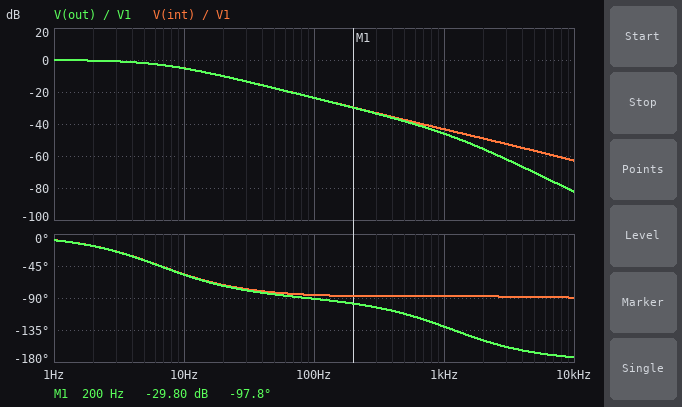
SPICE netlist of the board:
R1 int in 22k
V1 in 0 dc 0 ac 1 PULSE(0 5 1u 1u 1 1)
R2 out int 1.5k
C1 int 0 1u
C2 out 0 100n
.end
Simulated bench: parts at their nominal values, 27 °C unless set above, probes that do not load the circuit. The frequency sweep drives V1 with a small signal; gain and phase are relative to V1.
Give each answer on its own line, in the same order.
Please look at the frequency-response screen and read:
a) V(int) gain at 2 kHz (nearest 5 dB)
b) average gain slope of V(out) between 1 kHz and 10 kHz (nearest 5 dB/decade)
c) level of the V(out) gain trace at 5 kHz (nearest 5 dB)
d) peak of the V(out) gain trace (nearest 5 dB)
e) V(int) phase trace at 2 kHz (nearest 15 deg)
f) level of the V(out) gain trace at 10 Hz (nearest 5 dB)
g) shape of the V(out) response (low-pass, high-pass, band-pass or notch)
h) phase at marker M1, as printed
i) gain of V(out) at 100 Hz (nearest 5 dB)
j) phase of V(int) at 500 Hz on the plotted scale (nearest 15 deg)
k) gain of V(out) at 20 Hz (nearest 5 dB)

-50 dB
-35 dB/decade
-70 dB
0 dB
-90 deg
-5 dB
low-pass
-97.8 deg
-25 dB
-90 deg
-10 dB
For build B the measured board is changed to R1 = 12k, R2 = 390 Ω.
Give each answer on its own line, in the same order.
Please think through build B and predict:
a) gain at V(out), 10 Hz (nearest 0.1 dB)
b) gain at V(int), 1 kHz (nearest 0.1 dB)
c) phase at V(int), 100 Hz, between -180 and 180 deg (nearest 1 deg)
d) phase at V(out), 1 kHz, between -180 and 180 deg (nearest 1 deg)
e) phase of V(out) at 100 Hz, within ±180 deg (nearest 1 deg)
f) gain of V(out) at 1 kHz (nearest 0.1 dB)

-2.3 dB
-38.3 dB
-83 deg
-102 deg
-84 deg
-38.6 dB
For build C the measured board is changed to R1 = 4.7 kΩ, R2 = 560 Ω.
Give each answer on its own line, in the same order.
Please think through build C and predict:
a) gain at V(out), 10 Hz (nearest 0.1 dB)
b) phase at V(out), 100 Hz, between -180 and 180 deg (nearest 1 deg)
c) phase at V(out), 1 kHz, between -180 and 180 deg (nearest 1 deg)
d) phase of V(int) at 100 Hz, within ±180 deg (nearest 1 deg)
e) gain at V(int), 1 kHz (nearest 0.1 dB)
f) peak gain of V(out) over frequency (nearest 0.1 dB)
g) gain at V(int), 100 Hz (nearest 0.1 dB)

-0.4 dB
-75 deg
-106 deg
-73 deg
-30.2 dB
0 dB
-10.6 dB
